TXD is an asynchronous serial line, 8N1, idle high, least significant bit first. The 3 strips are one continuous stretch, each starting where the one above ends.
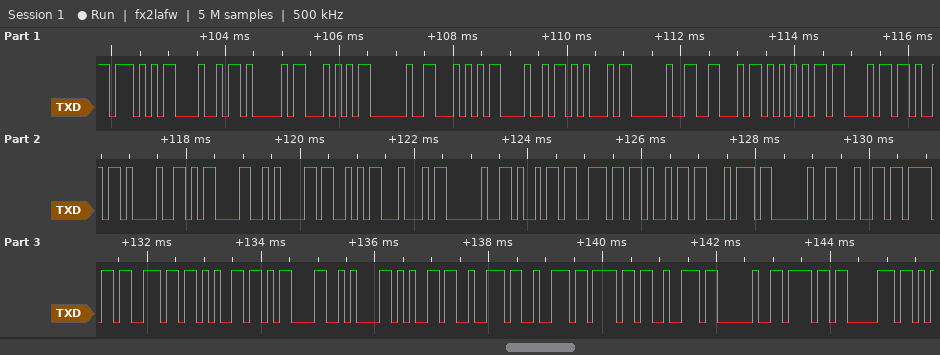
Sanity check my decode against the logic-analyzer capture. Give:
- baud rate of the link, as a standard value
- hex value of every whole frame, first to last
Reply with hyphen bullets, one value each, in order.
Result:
- 9600 baud
- 57 48 41 54 20 54 48 45 20 46 55 43 4B 21 0D 0A 53 44 20 69 6E 69 74 20 64 6F 6E 65 0D 0A 65 72 72 6F 72 20 6F 70
